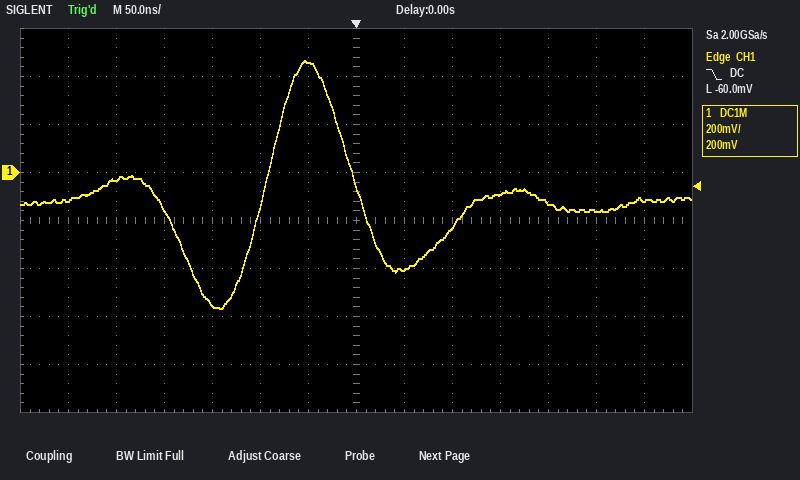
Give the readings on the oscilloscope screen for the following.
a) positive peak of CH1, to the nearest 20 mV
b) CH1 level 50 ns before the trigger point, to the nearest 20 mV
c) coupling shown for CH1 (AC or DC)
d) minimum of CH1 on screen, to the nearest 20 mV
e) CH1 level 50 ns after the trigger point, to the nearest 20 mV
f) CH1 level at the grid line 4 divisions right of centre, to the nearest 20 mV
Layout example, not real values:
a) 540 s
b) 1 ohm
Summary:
a) 460 mV
b) 460 mV
c) DC
d) -560 mV
e) -400 mV
f) -120 mV
